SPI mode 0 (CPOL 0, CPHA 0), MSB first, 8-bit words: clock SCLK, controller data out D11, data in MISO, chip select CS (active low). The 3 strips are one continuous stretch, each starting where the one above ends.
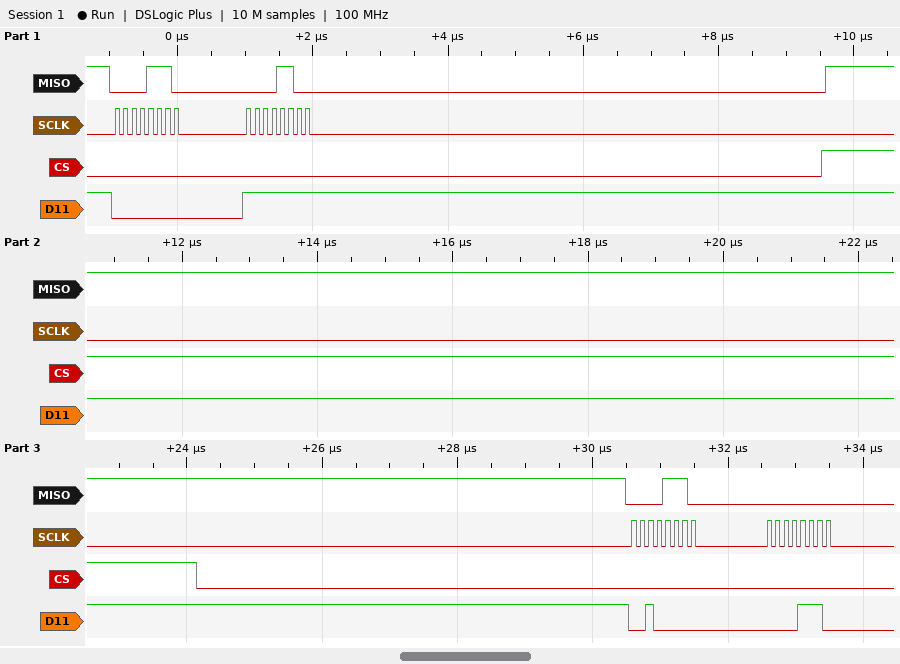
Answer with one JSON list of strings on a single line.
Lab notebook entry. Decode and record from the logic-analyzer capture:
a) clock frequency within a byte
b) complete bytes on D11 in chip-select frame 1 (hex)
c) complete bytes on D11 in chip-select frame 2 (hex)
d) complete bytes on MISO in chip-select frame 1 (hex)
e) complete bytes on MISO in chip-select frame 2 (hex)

["8 MHz", "0x00 0xFF", "0x20 0x0E", "0x0E 0x0C", "0x0E 0x00"]
